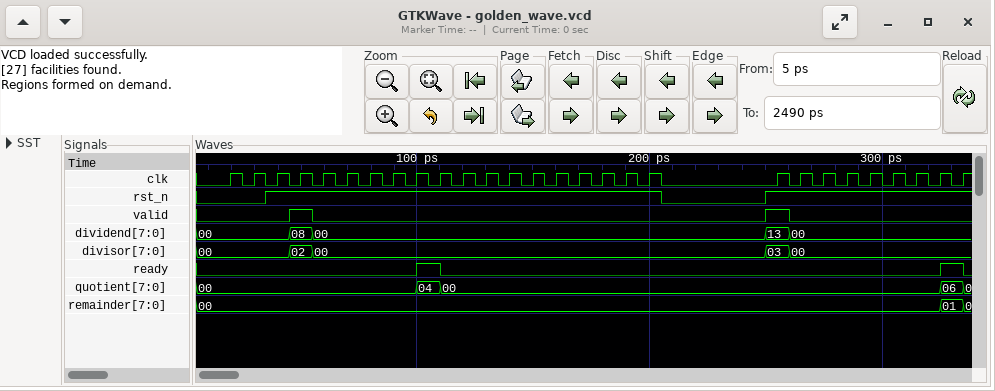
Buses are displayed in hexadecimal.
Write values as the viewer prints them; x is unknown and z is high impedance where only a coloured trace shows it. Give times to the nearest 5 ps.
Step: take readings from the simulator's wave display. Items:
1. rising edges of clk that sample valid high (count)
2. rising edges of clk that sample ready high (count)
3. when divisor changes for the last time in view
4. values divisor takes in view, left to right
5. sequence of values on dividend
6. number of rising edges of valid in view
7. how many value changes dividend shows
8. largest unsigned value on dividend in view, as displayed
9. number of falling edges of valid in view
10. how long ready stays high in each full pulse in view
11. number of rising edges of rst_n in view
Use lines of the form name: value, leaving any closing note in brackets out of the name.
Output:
rising edges of clk that sample valid high: 2
rising edges of clk that sample ready high: 2
when divisor changes for the last time in view: 260 ps
values divisor takes in view, left to right: 00, 02, 00, 03, 00
sequence of values on dividend: 00, 08, 00, 13, 00
number of rising edges of valid in view: 2
how many value changes dividend shows: 4
largest unsigned value on dividend in view, as displayed: 13
number of falling edges of valid in view: 2
how long ready stays high in each full pulse in view: 10 ps, 10 ps
number of rising edges of rst_n in view: 2
